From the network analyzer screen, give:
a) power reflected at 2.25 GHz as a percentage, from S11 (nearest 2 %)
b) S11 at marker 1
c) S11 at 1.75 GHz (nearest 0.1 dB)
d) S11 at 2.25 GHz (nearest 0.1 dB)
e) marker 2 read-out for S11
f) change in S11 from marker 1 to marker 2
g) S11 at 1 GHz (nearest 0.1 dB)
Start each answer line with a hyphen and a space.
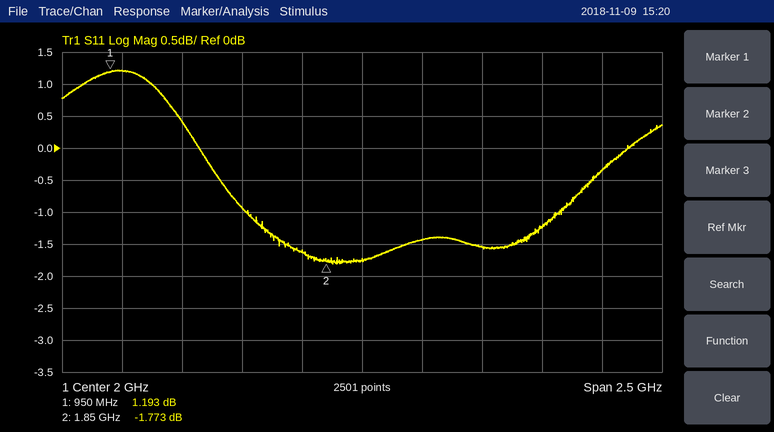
- 72 %
- 1.193 dB
- -1.6 dB
- -1.4 dB
- -1.773 dB
- -2.966 dB
- 1.2 dB
